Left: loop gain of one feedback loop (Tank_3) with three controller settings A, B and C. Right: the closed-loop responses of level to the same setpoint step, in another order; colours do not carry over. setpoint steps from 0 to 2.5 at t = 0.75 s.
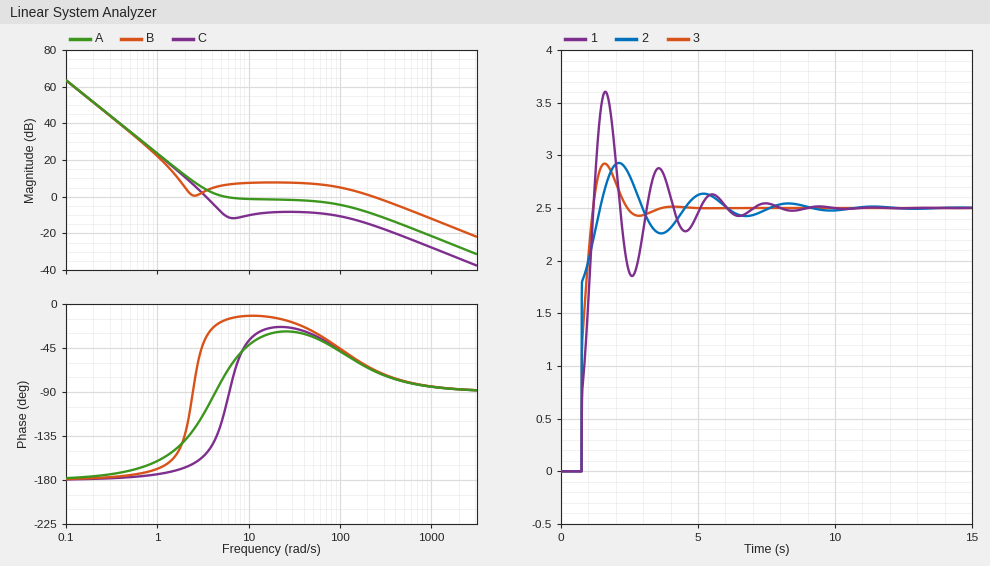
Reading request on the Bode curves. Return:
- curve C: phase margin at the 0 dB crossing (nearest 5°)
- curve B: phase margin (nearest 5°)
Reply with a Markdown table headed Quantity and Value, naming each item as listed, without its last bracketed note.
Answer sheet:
| Quantity | Value |
|---|---|
| curve C: phase margin at the 0 dB crossing | 25° |
| curve B: phase margin | 115° |
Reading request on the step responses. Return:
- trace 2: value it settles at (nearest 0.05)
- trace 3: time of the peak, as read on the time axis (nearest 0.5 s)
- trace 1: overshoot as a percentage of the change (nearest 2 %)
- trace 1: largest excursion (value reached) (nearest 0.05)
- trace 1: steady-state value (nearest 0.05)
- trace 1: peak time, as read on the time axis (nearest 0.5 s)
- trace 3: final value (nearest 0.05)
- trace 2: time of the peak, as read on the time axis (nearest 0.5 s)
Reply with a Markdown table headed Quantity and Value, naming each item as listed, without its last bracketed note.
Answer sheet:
| Quantity | Value |
|---|---|
| trace 2: value it settles at | 2.50 |
| trace 3: time of the peak, as read on the time axis | 1.5 s |
| trace 1: overshoot as a percentage of the change | 44 % |
| trace 1: largest excursion (value reached) | 3.60 |
| trace 1: steady-state value | 2.50 |
| trace 1: peak time, as read on the time axis | 1.5 s |
| trace 3: final value | 2.50 |
| trace 2: time of the peak, as read on the time axis | 2.0 s |
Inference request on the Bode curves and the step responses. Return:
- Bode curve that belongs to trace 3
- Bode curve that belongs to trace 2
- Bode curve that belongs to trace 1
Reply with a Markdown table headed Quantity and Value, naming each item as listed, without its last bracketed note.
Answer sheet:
| Quantity | Value |
|---|---|
| Bode curve that belongs to trace 3 | A |
| Bode curve that belongs to trace 2 | B |
| Bode curve that belongs to trace 1 | C |
